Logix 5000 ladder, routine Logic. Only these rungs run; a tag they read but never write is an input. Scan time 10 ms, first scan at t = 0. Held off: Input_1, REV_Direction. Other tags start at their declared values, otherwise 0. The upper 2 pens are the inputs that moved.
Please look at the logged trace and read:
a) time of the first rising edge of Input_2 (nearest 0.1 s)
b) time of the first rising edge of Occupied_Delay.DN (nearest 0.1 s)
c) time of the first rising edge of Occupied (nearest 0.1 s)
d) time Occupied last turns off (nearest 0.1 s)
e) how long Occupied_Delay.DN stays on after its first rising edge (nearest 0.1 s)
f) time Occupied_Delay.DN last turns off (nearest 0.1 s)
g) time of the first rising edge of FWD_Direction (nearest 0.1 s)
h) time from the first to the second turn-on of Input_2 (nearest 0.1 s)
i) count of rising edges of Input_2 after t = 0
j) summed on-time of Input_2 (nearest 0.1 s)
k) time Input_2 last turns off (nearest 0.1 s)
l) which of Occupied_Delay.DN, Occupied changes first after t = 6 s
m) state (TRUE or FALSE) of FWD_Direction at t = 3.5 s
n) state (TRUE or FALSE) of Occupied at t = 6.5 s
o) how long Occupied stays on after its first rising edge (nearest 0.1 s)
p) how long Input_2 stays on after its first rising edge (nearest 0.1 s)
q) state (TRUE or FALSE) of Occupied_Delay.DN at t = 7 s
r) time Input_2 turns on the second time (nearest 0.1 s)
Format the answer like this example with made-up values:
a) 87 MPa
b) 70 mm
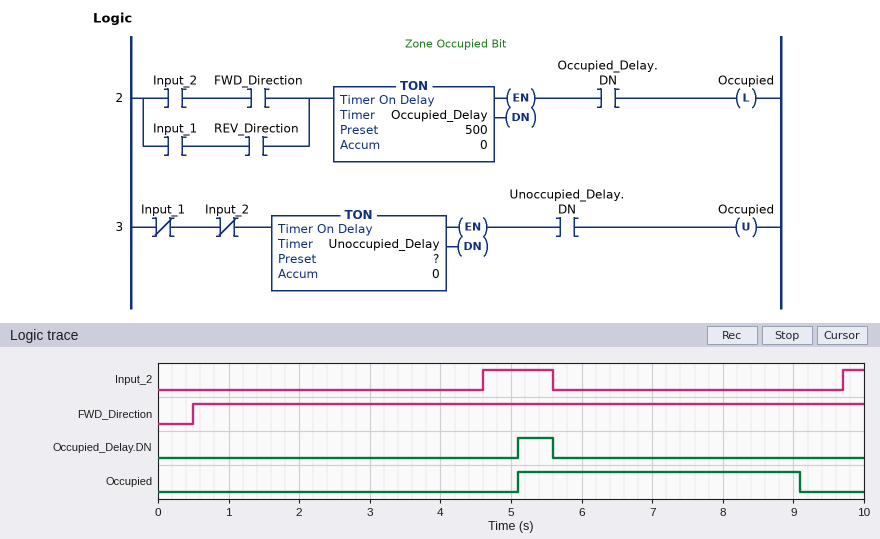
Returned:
a) 4.6 s
b) 5.1 s
c) 5.1 s
d) 9.1 s
e) 0.5 s
f) 5.6 s
g) 0.5 s
h) 5.1 s
i) 2
j) 1.3 s
k) 5.6 s
l) Occupied
m) TRUE
n) TRUE
o) 4.0 s
p) 1.0 s
q) FALSE
r) 9.7 s
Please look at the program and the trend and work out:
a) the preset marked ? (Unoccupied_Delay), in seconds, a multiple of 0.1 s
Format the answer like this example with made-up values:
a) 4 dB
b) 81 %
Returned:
a) 3.5 s
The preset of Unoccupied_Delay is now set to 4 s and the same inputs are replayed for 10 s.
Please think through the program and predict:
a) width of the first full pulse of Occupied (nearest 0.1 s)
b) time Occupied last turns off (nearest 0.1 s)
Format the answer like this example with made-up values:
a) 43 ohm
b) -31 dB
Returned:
a) 4.5 s
b) 9.6 s
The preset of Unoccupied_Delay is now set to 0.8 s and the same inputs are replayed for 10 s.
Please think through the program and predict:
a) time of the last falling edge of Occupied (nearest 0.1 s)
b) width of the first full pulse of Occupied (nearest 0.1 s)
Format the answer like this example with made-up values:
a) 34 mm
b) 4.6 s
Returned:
a) 6.4 s
b) 1.3 s
